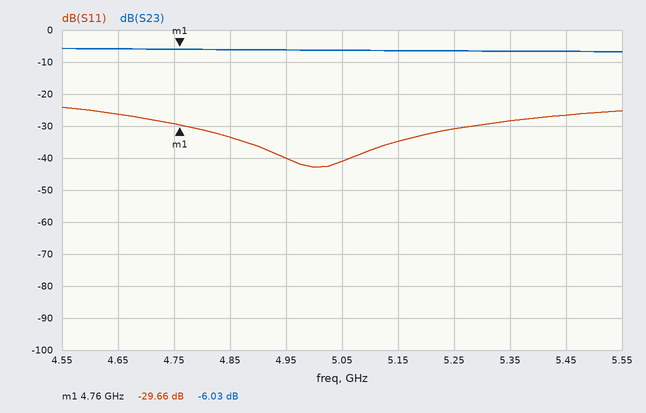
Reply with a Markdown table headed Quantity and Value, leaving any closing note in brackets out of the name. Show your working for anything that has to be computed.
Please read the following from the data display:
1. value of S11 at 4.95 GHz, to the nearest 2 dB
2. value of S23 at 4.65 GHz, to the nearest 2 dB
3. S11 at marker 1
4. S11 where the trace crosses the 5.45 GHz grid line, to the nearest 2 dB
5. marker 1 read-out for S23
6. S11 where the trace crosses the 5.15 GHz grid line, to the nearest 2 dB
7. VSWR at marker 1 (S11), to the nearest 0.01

| Quantity | Value |
|---|---|
| value of S11 at 4.95 GHz, to the nearest 2 dB | -40 dB |
| value of S23 at 4.65 GHz, to the nearest 2 dB | -6 dB |
| S11 at marker 1 | -29.66 dB |
| S11 where the trace crosses the 5.45 GHz grid line, to the nearest 2 dB | -26 dB |
| marker 1 read-out for S23 | -6.03 dB |
| S11 where the trace crosses the 5.15 GHz grid line, to the nearest 2 dB | -34 dB |
| VSWR at marker 1 (S11), to the nearest 0.01 | (1 + 0.0329)/(1 − 0.0329) ≈ 1.07 |
